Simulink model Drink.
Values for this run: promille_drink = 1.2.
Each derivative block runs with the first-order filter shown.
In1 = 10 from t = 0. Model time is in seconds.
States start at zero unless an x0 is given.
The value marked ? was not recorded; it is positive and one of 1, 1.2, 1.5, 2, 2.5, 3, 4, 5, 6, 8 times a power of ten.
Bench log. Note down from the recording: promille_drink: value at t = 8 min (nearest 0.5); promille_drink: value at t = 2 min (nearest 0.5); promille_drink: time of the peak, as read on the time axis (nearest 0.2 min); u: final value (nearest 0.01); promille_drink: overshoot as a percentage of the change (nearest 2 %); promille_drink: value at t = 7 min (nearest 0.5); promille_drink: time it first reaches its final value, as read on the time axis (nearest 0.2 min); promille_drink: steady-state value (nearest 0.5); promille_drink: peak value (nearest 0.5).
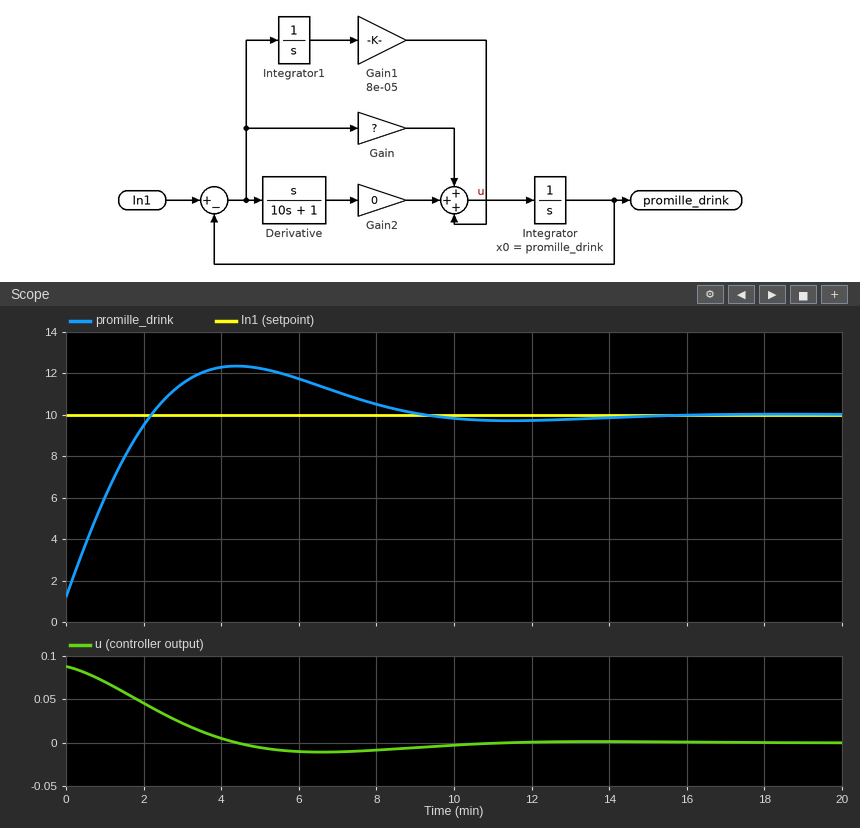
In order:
10.5
9.5
4.4 min
0.00
26 %
11.0
2.2 min
10.0
12.5
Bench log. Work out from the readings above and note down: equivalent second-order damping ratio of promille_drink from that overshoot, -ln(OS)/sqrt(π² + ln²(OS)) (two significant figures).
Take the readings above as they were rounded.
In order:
0.39
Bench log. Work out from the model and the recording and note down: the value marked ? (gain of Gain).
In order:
0.01
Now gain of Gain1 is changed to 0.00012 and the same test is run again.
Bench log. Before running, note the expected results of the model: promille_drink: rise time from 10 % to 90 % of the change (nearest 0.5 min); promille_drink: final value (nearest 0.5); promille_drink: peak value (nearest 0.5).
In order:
1.5 min
10.0
13.0
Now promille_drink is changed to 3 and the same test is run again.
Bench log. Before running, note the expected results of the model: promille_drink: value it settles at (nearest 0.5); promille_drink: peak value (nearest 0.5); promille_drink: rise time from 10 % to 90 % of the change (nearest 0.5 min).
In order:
10.0
12.0
1.5 min
